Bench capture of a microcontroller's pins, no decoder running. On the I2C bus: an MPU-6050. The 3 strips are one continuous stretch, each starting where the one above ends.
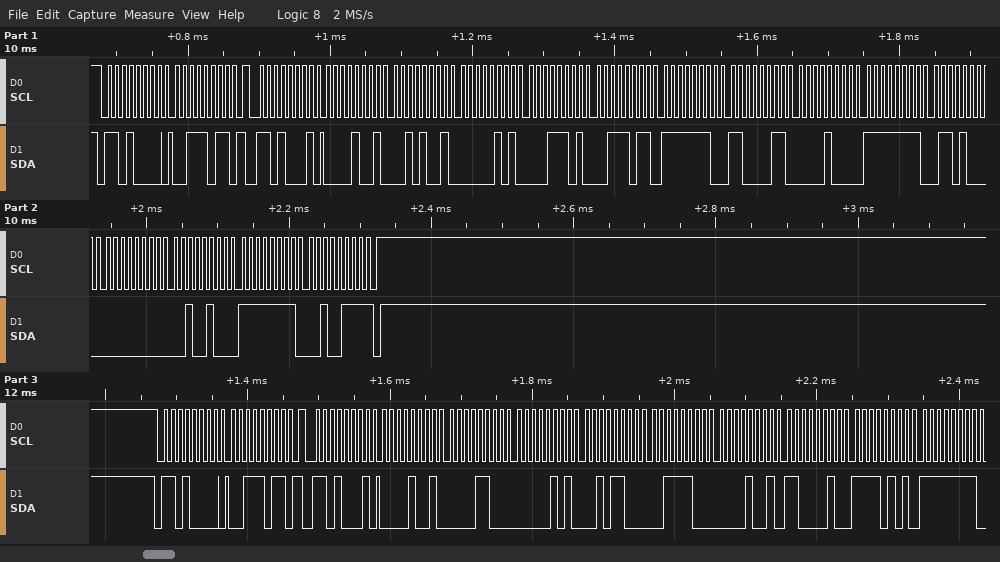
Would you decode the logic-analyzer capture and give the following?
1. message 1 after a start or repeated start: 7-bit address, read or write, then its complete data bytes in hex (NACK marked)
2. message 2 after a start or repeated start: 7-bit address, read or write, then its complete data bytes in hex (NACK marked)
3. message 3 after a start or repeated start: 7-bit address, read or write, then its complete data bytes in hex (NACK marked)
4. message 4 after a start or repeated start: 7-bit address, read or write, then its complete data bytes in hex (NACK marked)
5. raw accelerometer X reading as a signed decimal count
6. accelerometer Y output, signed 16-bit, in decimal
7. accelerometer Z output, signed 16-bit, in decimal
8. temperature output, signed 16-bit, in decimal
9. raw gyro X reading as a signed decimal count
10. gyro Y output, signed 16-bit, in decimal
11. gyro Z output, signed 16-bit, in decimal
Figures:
0x68 write: 3B
0x68 read: 09 29 05 1D 3B FE C3 08 FF 68 00 24 FF 27 NACK
0x68 write: 3B
0x68 read: 09 0C 05 2C 3C 09 C2 F5 FF
2345
1309
15358
-15608
-152
36
-217
